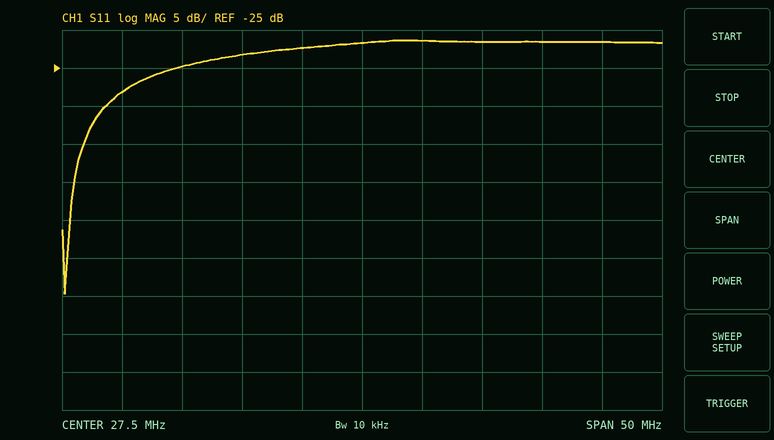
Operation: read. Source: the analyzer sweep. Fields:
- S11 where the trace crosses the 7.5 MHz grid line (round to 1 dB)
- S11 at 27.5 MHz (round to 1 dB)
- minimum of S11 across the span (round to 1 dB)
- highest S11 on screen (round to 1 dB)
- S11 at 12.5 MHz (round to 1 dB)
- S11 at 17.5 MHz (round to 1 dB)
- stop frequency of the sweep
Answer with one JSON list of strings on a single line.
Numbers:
["-28 dB", "-22 dB", "-55 dB", "-21 dB", "-25 dB", "-23 dB", "52.5 MHz"]
